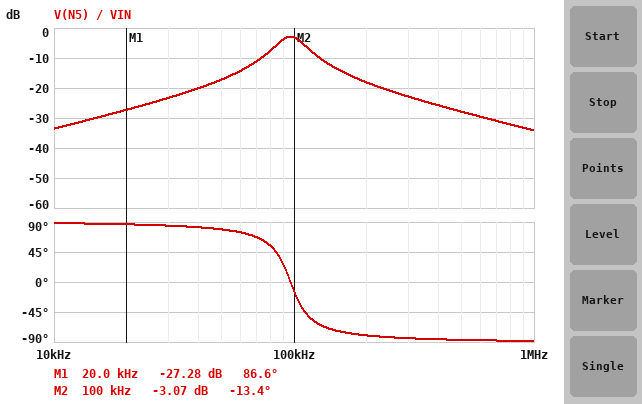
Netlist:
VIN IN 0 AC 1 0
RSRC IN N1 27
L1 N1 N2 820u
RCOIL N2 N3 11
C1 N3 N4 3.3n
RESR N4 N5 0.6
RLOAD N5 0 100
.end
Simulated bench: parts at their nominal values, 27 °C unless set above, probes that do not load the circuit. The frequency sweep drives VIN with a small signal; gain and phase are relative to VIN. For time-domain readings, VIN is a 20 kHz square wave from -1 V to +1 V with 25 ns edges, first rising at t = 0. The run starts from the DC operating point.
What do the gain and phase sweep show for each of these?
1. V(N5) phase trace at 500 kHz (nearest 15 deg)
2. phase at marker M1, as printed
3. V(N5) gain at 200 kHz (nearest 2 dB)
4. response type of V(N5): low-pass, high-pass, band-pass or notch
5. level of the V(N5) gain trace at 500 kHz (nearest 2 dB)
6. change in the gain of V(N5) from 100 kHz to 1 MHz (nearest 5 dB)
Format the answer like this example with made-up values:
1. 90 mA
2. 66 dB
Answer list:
1. -90 deg
2. 86.6 deg
3. -18 dB
4. band-pass
5. -28 dB
6. -30 dB
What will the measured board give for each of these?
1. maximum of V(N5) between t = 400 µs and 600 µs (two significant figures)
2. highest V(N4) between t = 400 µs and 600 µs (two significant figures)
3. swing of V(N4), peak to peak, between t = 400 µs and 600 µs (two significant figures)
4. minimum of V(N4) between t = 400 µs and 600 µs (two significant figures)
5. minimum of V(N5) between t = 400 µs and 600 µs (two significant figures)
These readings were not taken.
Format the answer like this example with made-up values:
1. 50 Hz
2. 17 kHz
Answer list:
1. 360 mV
2. 360 mV
3. 720 mV
4. -360 mV
5. -360 mV
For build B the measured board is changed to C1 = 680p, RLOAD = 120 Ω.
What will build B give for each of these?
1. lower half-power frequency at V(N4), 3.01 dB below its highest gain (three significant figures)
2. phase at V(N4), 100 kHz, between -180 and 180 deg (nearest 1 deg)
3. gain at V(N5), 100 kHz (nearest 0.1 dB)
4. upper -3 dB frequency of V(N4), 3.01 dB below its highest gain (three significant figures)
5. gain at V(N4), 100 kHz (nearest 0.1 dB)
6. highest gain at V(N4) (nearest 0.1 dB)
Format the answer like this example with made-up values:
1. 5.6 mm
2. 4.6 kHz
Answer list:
1. 198 kHz
2. 85 deg
3. -23.7 dB
4. 229 kHz
5. -23.6 dB
6. -2.4 dB
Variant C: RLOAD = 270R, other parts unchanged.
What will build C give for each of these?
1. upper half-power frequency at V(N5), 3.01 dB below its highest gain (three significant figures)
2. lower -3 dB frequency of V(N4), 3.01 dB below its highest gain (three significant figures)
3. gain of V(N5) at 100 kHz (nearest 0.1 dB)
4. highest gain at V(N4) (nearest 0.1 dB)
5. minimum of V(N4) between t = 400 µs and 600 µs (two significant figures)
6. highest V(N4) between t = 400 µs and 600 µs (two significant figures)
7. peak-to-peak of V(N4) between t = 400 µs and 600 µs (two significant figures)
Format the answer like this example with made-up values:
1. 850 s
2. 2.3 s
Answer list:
1. 131 kHz
2. 71.3 kHz
3. -1.2 dB
4. -1.1 dB
5. -720 mV
6. 720 mV
7. 1.4 V
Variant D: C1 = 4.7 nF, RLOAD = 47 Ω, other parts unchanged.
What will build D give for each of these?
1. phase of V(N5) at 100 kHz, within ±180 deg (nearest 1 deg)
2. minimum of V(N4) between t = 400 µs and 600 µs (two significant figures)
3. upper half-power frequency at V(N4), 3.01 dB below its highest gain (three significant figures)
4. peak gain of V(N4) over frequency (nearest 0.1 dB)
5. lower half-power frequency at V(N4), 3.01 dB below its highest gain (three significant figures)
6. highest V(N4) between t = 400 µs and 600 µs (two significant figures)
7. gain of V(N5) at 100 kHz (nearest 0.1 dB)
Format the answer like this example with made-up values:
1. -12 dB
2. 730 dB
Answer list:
1. -64 deg
2. -150 mV
3. 89.8 kHz
4. -5.1 dB
5. 73.2 kHz
6. 150 mV
7. -12.4 dB
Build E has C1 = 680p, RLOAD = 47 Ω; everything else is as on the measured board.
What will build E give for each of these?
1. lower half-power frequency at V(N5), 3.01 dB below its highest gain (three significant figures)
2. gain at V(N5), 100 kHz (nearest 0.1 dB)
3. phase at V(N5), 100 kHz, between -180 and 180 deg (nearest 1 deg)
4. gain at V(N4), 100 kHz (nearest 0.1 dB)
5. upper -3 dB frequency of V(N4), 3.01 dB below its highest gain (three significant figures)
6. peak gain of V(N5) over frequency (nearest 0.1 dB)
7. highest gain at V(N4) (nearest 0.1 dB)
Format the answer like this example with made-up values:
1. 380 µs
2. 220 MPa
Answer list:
1. 205 kHz
2. -31.8 dB
3. 87 deg
4. -31.7 dB
5. 222 kHz
6. -5.2 dB
7. -5.1 dB
